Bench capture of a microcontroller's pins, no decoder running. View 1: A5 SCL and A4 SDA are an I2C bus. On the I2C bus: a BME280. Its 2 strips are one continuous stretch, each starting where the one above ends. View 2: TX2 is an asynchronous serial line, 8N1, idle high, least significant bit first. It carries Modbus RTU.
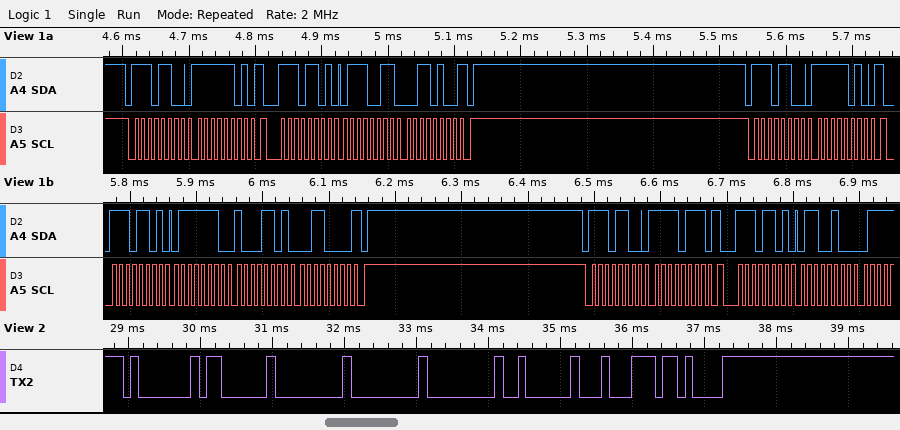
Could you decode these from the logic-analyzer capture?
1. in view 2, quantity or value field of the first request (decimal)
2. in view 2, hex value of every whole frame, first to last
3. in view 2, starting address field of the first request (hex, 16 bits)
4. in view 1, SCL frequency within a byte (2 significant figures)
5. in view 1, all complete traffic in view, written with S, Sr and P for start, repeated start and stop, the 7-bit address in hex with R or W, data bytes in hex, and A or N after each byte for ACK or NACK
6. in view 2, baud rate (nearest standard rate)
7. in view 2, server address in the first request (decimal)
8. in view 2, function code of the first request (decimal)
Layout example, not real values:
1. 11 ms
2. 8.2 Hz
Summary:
1. 2
2. 01 03 00 00 00 02 C4 0B
3. 0x0000
4. 100 kHz
5. S 76W A FD A Sr 76R A 73 A 34 N P S 76W A FA A Sr 76R A 7E A 8D A 30 N P S 76W A F7 A Sr 76R A 64 A
6. 9600 baud
7. 1
8. 3
